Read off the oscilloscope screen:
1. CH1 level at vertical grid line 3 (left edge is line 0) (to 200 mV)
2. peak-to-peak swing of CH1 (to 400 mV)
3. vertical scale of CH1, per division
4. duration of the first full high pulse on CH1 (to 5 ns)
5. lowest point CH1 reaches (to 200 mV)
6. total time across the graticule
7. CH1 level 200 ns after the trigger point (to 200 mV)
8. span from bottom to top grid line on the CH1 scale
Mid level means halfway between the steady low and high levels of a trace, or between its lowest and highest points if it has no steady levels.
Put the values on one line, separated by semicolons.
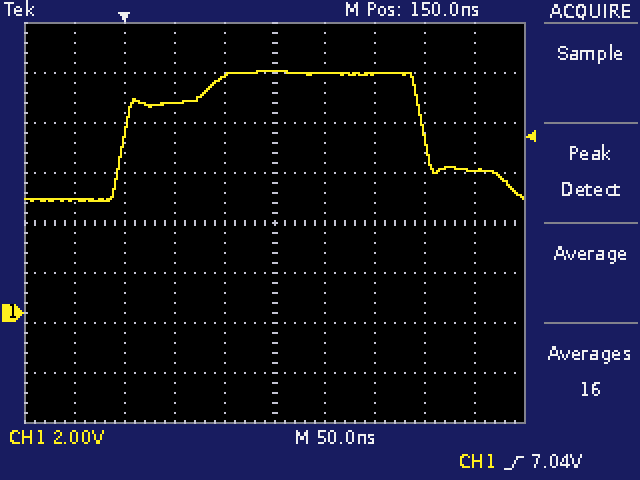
8.4 V; 5.2 V; 2 V; 300 ns; 4.4 V; 500 ns; 9.6 V; 16 V
